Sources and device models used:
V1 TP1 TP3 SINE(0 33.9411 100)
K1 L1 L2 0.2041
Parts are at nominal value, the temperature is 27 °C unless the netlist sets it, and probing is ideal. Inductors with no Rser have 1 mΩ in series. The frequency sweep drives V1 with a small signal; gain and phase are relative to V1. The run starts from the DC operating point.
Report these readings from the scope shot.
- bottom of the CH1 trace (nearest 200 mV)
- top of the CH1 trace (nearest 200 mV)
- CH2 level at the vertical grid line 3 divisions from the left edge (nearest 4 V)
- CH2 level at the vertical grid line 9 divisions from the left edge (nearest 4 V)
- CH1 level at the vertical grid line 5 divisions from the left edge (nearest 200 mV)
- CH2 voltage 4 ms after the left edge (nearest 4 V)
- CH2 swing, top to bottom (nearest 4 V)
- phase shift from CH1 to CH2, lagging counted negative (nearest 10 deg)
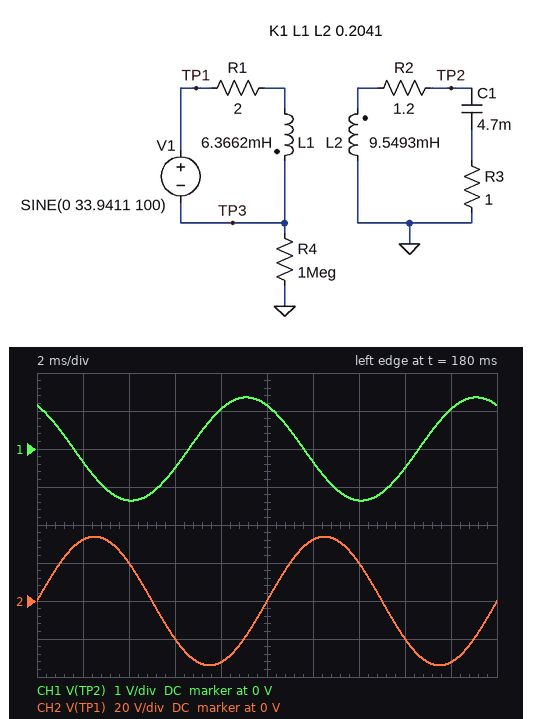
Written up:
-1.4 V
1.4 V
-20 V
-32 V
1.2 V
20 V
68 V
-120 deg
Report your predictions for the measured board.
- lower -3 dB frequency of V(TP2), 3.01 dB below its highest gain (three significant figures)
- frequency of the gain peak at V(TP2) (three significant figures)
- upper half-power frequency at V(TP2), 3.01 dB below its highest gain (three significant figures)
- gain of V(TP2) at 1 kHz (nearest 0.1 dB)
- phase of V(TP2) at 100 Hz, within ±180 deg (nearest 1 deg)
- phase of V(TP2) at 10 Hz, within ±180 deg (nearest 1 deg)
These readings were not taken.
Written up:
12.3 Hz
28.8 Hz
69.0 Hz
-47.2 dB
122 deg
-127 deg
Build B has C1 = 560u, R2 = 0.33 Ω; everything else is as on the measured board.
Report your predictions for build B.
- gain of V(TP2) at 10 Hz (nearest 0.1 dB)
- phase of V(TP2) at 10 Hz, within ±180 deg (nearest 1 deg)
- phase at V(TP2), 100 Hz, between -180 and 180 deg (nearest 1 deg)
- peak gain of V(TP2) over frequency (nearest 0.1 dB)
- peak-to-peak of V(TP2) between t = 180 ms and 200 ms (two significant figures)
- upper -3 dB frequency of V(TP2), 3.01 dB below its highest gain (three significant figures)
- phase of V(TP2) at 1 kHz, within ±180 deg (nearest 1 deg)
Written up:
-26.3 dB
-107 deg
92 deg
-8.1 dB
19 V
99.9 Hz
78 deg
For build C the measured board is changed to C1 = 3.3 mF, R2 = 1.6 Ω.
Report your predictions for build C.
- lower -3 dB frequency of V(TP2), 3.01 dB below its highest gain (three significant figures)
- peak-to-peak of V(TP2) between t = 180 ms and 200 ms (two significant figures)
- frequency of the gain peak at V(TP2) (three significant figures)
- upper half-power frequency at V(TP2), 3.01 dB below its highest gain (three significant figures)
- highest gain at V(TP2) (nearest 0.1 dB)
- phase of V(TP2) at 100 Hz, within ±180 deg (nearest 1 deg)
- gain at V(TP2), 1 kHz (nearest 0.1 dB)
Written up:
12.9 Hz
2.8 V
29.7 Hz
68.1 Hz
-22.0 dB
121 deg
-47.2 dB
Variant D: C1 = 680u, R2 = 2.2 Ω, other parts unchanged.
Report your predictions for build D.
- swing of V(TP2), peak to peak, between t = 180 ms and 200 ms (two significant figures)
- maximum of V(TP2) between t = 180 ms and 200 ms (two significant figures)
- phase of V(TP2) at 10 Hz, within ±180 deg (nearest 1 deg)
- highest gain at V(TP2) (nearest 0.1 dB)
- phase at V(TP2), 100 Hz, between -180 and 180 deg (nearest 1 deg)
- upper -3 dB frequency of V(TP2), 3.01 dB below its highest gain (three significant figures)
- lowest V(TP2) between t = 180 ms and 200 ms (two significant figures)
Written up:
7.6 V
3.8 V
-112 deg
-15.8 dB
107 deg
98.3 Hz
-3.8 V
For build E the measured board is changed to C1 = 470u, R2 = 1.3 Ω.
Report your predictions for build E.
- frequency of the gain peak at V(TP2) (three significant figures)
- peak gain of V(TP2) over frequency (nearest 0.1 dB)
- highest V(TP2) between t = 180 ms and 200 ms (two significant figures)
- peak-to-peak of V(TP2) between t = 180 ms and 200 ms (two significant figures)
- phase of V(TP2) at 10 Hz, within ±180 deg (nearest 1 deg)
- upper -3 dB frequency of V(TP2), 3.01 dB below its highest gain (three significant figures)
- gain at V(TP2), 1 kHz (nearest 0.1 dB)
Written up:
85.4 Hz
-11.7 dB
7.9 V
16 V
-109 deg
114 Hz
-46.7 dB
